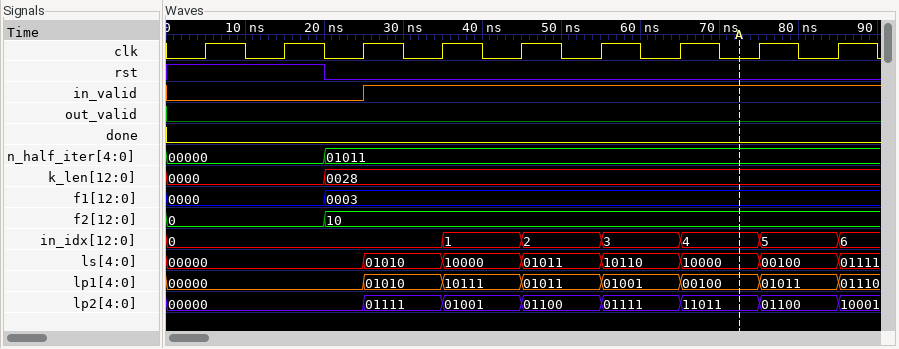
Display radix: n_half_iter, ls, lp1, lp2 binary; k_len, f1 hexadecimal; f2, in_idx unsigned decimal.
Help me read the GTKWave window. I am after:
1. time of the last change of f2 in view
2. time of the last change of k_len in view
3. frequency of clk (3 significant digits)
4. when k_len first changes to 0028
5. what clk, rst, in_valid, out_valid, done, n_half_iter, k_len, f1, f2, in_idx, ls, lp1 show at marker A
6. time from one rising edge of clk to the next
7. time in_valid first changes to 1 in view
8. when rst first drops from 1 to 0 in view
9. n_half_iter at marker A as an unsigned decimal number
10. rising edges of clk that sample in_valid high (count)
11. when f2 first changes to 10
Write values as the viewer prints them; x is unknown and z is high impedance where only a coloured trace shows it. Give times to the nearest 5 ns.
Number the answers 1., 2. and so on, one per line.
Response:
1. 20 ns
2. 20 ns
3. 100 MHz
4. 20 ns
5. clk=0, rst=0, in_valid=1, out_valid=0, done=0, n_half_iter=01011, k_len=0028, f1=0003, f2=10, in_idx=4, ls=10000, lp1=00100
6. 10 ns
7. 25 ns
8. 20 ns
9. 11
10. 6
11. 20 ns
